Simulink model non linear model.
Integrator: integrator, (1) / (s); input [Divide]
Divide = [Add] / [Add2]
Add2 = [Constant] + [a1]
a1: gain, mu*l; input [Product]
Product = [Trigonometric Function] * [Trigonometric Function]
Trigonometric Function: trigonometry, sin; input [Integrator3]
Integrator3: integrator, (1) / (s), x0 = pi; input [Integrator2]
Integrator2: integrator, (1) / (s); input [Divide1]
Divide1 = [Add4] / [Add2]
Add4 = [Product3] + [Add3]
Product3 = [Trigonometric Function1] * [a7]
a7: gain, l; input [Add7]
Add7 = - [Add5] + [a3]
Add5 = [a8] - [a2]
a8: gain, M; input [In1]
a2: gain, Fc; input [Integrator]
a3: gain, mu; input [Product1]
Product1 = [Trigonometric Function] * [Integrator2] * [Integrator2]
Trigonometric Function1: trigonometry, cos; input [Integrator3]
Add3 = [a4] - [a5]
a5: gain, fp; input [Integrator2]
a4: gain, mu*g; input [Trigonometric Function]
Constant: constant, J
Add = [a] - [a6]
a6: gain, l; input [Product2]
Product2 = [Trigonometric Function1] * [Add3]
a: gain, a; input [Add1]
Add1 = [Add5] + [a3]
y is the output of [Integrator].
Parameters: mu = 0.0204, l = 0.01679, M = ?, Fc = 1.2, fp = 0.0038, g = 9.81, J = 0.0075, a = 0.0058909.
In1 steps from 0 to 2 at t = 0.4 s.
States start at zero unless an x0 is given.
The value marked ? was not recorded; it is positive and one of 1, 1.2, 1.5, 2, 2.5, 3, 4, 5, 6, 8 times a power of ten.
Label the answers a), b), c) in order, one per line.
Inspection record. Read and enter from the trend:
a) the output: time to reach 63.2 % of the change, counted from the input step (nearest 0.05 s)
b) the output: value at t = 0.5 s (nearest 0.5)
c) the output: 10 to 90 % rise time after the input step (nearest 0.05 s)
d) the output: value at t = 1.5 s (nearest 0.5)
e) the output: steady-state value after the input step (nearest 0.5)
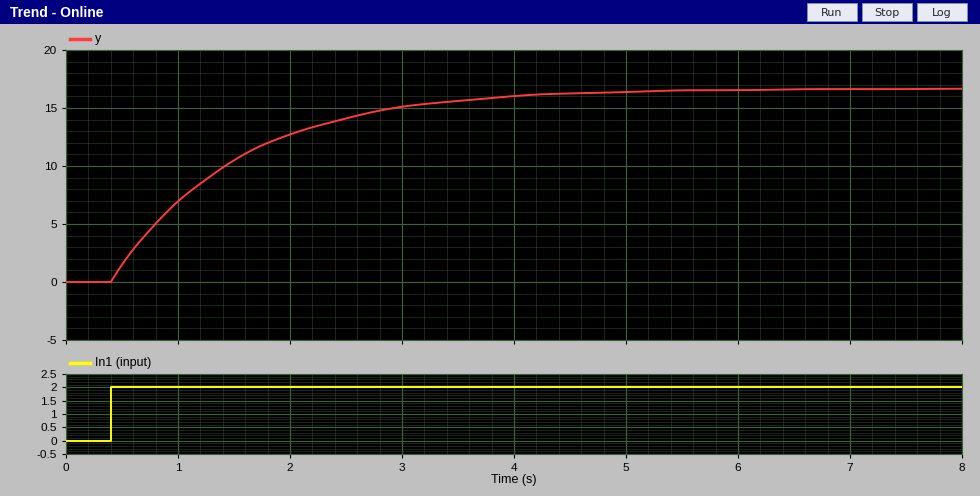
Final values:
a) 1.10 s
b) 1.5
c) 2.40 s
d) 10.5
e) 16.5
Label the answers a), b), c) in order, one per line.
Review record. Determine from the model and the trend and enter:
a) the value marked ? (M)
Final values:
a) 10
